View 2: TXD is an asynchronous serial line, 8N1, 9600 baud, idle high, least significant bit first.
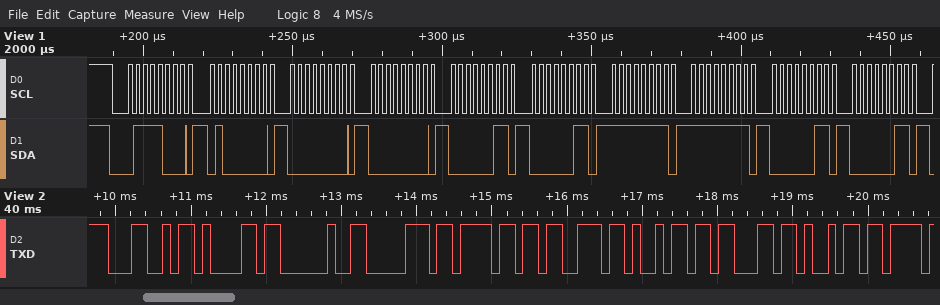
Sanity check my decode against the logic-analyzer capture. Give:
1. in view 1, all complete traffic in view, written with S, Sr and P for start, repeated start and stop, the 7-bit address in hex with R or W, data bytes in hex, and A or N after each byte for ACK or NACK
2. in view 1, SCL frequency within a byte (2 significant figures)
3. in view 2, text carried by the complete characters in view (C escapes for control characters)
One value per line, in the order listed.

S 3CW A 40 A 00 A 00 A 03 A 03 A FF A FF A 03 A 03 A
400 kHz
"La posici"
